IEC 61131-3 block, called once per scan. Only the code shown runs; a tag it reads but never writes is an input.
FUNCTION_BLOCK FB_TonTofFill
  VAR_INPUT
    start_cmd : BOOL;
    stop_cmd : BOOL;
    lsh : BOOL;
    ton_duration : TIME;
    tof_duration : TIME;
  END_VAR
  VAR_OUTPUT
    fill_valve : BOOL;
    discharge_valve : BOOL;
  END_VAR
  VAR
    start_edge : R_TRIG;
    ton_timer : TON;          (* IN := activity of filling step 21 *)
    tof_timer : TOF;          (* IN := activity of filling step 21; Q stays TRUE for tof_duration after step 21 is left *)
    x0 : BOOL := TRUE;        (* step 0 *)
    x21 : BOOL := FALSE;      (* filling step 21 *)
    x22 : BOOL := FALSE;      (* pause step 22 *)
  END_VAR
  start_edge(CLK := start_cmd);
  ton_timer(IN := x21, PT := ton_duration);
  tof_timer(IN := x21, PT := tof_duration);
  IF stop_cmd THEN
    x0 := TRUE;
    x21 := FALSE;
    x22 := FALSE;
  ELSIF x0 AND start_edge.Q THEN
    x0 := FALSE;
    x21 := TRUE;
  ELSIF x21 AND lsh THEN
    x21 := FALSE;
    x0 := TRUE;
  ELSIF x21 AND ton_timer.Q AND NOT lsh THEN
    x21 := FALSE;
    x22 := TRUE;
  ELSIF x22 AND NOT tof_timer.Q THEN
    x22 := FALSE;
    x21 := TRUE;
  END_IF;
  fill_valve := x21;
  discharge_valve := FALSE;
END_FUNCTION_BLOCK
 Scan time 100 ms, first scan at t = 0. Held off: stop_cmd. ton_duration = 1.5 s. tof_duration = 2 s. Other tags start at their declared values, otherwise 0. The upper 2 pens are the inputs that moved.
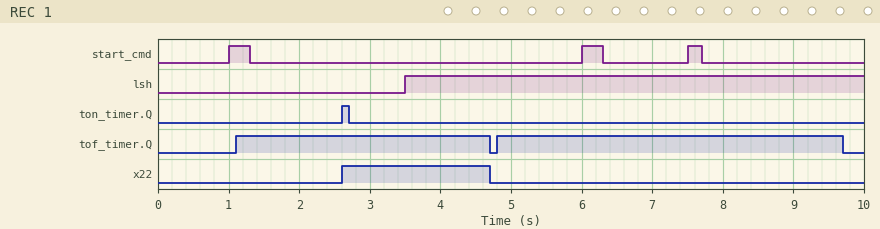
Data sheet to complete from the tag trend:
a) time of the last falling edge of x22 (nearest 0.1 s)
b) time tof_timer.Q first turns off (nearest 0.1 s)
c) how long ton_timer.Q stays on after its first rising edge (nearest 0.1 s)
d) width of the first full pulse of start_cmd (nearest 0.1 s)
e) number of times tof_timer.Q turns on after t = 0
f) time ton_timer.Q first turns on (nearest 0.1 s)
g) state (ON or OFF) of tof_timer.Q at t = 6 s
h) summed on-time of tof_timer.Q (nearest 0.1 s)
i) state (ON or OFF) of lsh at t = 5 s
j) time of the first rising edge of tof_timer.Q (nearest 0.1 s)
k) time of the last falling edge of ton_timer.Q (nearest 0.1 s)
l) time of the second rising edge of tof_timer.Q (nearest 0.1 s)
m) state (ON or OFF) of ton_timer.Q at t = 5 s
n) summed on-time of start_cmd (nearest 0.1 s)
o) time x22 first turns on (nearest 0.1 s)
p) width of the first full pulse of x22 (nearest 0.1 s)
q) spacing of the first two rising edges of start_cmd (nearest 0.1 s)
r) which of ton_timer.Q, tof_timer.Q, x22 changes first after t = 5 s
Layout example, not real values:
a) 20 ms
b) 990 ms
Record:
a) 4.7 s
b) 4.7 s
c) 0.1 s
d) 0.3 s
e) 2
f) 2.6 s
g) ON
h) 8.5 s
i) ON
j) 1.1 s
k) 2.7 s
l) 4.8 s
m) OFF
n) 0.8 s
o) 2.6 s
p) 2.1 s
q) 5.0 s
r) tof_timer.Q
